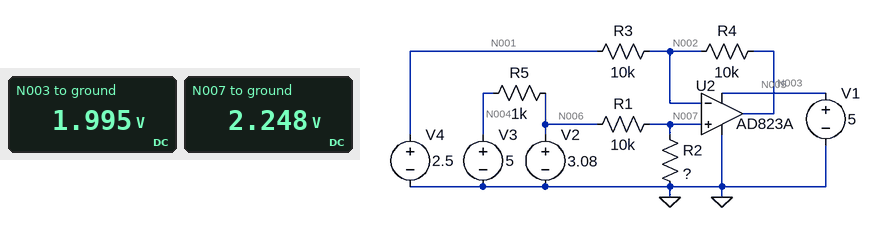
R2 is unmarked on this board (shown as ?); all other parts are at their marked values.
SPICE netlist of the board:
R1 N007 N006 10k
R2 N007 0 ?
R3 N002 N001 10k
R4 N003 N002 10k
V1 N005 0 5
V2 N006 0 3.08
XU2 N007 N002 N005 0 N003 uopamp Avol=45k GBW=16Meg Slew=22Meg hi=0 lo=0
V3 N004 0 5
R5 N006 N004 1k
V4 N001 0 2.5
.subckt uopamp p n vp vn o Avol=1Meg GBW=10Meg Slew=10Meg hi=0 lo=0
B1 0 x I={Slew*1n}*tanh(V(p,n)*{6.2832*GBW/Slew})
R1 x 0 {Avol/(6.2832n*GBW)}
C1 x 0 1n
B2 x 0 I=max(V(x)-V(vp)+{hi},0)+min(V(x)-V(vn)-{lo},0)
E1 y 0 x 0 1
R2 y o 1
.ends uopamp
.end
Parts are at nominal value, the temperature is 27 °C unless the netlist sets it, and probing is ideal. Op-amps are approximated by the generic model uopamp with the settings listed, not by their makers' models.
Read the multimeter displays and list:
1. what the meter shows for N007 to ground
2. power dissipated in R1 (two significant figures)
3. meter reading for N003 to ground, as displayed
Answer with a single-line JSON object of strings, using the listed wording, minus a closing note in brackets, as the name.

{"what the meter shows for N007 to ground": "2.248 V", "power dissipated in R1": "69 µW", "meter reading for N003 to ground, as displayed": "1.995 V"}
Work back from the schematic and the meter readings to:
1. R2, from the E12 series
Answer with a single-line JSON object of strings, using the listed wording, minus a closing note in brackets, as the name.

{"R2, from the E12 series": "27 kΩ"}
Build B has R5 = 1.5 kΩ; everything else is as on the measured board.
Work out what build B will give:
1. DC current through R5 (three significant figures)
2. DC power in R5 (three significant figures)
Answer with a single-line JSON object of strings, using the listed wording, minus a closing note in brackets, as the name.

{"DC current through R5": "1.28 mA", "DC power in R5": "2.46 mW"}
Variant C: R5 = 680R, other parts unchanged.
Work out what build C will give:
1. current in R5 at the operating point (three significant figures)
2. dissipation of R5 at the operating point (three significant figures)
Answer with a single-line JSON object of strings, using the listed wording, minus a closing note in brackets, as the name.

{"current in R5 at the operating point": "2.82 mA", "dissipation of R5 at the operating point": "5.42 mW"}
